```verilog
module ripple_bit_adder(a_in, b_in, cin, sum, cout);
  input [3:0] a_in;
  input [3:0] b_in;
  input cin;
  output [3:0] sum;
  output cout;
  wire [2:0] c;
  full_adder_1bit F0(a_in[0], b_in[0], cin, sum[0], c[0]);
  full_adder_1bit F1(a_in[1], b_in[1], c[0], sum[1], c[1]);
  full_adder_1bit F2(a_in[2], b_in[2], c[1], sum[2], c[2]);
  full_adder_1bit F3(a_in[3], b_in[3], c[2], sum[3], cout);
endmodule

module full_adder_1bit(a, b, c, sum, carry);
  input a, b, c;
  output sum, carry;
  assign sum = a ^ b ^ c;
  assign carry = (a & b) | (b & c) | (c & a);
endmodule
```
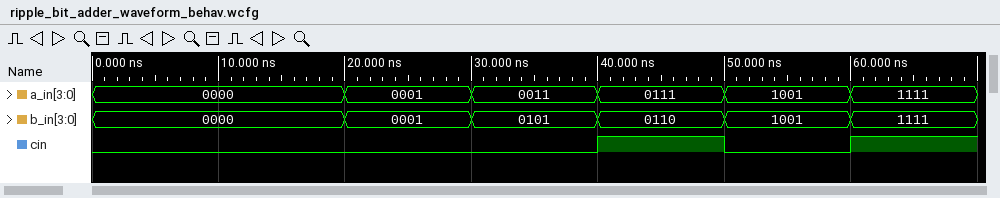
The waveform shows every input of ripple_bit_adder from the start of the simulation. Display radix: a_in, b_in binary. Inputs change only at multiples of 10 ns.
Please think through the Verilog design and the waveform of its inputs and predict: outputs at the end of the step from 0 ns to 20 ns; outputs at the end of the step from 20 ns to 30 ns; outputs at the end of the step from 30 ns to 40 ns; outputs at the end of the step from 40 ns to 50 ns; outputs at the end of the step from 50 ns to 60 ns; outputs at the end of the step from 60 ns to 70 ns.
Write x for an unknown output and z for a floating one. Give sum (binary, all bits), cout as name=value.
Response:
sum=0000, cout=0
sum=0010, cout=0
sum=1000, cout=0
sum=1110, cout=0
sum=0010, cout=1
sum=1111, cout=1
